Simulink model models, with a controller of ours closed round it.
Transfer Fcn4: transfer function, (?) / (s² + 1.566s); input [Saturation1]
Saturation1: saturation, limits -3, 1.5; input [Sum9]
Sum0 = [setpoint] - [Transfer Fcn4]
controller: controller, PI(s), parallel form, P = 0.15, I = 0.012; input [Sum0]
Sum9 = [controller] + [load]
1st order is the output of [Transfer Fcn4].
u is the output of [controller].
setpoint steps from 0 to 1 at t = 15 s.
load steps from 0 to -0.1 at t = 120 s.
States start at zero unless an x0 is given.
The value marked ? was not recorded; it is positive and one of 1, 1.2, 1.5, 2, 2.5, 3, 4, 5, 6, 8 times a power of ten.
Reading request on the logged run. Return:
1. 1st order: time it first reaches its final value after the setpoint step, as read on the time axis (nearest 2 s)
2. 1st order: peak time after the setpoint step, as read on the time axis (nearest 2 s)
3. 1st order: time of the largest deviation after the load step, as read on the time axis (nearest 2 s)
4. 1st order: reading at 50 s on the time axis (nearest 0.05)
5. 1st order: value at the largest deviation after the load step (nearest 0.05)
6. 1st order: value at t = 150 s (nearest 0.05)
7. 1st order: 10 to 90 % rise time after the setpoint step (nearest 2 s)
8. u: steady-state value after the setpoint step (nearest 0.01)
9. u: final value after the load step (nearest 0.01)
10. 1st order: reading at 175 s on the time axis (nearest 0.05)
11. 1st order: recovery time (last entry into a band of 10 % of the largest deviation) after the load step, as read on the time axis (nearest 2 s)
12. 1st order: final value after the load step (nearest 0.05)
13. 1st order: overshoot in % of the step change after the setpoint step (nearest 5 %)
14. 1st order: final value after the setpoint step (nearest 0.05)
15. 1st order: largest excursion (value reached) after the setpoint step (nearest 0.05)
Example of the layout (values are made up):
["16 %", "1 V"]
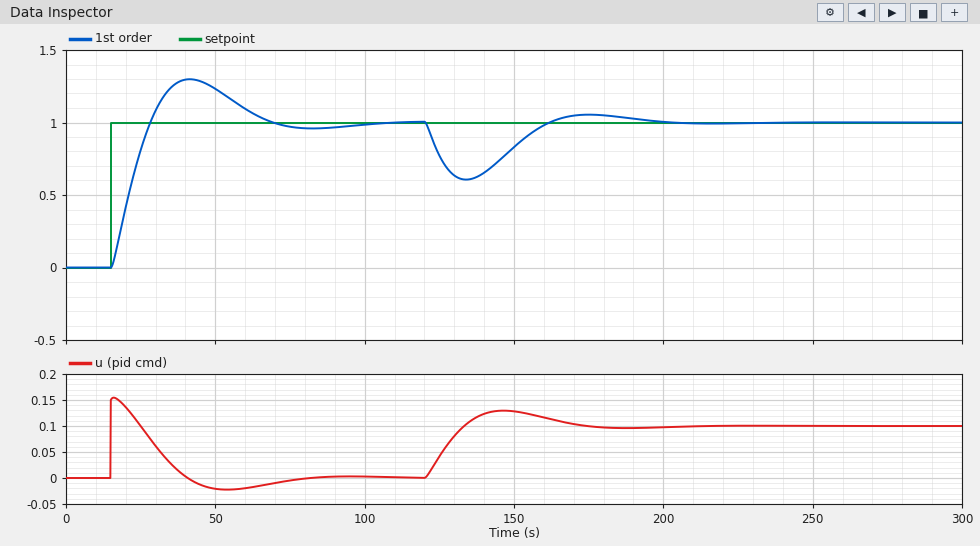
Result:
["28 s", "42 s", "134 s", "1.25", "0.60", "0.85", "10 s", "0.00", "0.10", "1.05", "184 s", "1.00", "30 %", "1.00", "1.30"]
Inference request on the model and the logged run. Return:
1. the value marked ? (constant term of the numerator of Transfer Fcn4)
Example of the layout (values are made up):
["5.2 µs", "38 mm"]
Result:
["1"]
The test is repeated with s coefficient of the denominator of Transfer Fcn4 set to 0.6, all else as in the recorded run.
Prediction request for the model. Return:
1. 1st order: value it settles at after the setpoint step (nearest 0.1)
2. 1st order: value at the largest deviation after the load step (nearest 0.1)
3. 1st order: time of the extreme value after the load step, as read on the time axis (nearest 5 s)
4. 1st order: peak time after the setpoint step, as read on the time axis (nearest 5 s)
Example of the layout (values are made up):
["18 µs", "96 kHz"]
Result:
["1.0", "0.4", "130 s", "25 s"]
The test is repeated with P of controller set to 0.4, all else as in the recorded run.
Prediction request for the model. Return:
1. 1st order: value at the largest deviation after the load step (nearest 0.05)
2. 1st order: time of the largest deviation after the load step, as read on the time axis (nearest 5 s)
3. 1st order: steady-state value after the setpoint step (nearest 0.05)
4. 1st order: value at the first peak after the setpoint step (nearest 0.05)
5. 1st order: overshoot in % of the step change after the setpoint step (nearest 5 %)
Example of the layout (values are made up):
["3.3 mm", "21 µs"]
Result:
["0.80", "130 s", "1.00", "1.10", "10 %"]
